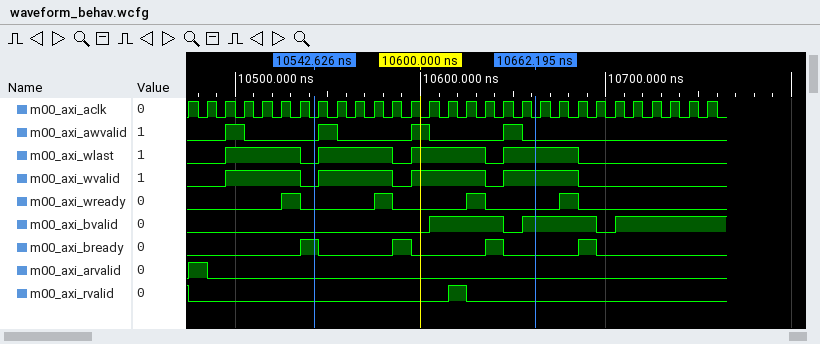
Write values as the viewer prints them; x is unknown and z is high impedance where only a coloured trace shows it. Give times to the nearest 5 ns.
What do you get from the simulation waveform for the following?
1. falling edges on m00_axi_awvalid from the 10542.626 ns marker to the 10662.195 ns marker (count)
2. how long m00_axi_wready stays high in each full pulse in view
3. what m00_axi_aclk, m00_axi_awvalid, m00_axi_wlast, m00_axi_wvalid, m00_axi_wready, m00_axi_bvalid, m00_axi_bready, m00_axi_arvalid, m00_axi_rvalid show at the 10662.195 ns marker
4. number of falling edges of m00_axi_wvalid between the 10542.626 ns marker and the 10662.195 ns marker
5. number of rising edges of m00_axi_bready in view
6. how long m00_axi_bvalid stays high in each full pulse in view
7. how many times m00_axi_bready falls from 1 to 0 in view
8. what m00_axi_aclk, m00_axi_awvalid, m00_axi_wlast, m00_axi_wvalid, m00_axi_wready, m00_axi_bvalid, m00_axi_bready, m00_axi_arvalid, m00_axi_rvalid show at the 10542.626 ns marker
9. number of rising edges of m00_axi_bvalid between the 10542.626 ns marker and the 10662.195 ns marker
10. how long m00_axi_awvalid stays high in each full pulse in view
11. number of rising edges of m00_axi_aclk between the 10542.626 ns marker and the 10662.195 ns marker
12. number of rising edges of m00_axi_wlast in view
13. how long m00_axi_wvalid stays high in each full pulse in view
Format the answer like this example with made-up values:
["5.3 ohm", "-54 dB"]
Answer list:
["3", "10 ns, 10 ns, 10 ns, 10 ns", "m00_axi_aclk=0, m00_axi_awvalid=0, m00_axi_wlast=1, m00_axi_wvalid=1, m00_axi_wready=0, m00_axi_bvalid=1, m00_axi_bready=0, m00_axi_arvalid=0, m00_axi_rvalid=0", "2", "4", "40 ns, 40 ns", "4", "m00_axi_aclk=0, m00_axi_awvalid=0, m00_axi_wlast=0, m00_axi_wvalid=0, m00_axi_wready=0, m00_axi_bvalid=0, m00_axi_bready=1, m00_axi_arvalid=0, m00_axi_rvalid=0", "2", "10 ns, 10 ns, 10 ns, 10 ns", "12", "4", "40 ns, 40 ns, 40 ns, 40 ns"]
